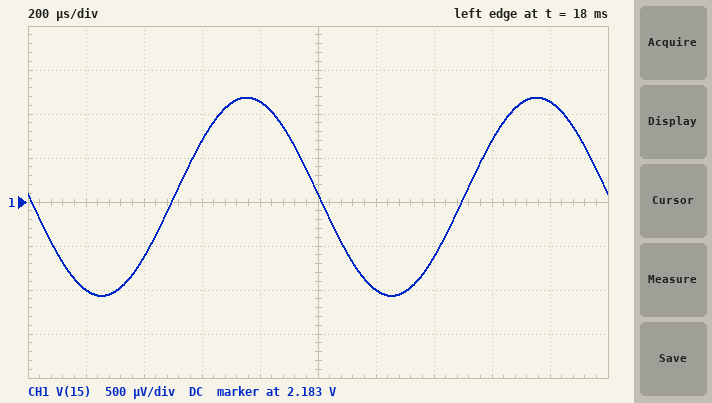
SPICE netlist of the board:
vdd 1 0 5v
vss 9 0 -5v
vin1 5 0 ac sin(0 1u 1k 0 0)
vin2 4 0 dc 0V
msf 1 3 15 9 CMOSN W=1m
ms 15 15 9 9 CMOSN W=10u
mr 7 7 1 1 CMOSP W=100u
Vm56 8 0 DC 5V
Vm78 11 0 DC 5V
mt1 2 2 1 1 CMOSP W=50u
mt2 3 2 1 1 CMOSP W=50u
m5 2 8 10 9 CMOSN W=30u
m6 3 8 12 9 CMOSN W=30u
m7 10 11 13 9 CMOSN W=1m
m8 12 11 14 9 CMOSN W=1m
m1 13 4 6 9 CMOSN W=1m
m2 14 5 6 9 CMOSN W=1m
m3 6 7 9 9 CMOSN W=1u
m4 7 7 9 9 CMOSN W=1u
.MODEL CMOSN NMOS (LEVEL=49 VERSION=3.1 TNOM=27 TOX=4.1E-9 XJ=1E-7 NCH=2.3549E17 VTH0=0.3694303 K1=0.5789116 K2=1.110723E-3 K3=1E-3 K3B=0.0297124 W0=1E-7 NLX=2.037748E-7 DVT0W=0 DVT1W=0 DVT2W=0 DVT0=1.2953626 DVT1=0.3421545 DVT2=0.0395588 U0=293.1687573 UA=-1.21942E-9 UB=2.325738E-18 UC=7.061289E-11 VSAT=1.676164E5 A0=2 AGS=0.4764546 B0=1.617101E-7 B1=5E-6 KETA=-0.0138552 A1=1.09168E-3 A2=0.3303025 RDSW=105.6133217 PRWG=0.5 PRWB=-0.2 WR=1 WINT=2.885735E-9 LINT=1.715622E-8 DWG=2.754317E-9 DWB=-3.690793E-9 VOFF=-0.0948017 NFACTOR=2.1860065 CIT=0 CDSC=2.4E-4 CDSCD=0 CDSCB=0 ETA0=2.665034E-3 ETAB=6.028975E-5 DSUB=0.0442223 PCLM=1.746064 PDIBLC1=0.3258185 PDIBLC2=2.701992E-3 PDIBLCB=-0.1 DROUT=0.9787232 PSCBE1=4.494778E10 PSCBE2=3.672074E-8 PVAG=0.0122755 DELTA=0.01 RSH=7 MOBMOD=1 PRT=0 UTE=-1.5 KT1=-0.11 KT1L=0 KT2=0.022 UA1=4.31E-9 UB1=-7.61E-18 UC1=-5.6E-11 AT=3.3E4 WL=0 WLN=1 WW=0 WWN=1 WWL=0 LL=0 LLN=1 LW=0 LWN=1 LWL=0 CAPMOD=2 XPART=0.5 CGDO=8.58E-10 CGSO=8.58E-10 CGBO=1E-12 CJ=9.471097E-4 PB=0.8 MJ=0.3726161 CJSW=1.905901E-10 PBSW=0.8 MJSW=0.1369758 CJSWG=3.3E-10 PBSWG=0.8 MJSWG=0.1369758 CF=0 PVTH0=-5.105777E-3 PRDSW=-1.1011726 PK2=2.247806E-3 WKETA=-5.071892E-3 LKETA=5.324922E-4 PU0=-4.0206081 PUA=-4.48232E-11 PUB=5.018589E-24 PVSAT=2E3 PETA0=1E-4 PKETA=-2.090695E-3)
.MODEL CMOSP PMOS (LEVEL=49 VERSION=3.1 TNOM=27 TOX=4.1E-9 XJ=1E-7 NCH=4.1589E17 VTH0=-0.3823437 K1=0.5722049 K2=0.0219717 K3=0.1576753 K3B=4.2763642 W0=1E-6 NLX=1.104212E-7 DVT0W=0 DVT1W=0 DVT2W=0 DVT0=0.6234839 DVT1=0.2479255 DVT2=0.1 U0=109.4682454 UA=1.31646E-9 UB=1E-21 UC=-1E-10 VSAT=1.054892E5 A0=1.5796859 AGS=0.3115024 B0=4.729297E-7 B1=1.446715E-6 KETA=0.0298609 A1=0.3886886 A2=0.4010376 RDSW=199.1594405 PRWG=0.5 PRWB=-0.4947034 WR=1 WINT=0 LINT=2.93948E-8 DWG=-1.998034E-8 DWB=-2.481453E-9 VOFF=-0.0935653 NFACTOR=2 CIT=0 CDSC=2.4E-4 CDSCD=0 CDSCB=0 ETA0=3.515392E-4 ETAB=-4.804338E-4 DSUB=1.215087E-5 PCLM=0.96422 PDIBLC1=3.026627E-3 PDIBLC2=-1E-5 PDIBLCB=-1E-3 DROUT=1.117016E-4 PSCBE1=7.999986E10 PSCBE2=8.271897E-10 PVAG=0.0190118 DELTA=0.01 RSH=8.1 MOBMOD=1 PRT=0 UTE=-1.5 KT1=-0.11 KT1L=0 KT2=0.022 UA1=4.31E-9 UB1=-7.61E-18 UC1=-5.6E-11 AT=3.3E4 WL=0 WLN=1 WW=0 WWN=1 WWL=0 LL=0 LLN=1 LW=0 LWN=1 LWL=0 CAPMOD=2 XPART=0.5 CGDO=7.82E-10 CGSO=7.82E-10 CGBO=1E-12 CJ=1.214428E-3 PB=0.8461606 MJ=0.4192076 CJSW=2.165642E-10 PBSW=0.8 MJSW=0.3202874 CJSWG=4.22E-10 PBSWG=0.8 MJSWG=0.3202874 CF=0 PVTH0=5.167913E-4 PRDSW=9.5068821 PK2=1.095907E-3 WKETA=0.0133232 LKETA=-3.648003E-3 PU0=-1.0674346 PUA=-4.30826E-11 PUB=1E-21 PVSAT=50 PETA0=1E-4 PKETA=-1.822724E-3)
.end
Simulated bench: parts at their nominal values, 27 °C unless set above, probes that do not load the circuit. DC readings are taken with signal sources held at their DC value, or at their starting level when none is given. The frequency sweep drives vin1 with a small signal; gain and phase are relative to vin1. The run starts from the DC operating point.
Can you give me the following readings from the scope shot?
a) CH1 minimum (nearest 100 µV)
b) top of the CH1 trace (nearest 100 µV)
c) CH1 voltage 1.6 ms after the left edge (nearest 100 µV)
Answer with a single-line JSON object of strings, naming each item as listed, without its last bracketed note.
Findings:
{"CH1 minimum": "2.1819 V", "top of the CH1 trace": "2.1842 V", "CH1 voltage 1.6 ms after the left edge": "2.1837 V"}
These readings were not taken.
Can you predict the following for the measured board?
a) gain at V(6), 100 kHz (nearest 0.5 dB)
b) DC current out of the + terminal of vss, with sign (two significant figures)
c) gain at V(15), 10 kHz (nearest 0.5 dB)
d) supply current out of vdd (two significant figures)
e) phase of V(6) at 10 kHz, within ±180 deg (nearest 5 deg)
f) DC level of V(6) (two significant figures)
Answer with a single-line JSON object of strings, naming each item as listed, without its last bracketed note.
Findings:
{"gain at V(6), 100 kHz": "-7.0 dB", "DC current out of the + terminal of vss, with sign": "-3.8 mA", "gain at V(15), 10 kHz": "60.5 dB", "supply current out of vdd": "3.8 mA", "phase of V(6) at 10 kHz, within ±180 deg": "0 deg", "DC level of V(6)": "-1.1 V"}
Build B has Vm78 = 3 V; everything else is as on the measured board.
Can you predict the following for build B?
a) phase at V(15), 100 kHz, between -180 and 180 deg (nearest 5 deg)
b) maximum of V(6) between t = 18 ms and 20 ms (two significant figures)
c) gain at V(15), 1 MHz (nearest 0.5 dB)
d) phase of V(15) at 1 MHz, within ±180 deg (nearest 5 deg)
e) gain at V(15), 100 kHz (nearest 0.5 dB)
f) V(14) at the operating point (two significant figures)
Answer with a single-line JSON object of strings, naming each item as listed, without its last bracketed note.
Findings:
{"phase at V(15), 100 kHz, between -180 and 180 deg": "110 deg", "maximum of V(6) between t = 18 ms and 20 ms": "-1.1 V", "gain at V(15), 1 MHz": "32.0 dB", "phase of V(15) at 1 MHz, within ±180 deg": "80 deg", "gain at V(15), 100 kHz": "51.5 dB", "V(14) at the operating point": "1.6 V"}
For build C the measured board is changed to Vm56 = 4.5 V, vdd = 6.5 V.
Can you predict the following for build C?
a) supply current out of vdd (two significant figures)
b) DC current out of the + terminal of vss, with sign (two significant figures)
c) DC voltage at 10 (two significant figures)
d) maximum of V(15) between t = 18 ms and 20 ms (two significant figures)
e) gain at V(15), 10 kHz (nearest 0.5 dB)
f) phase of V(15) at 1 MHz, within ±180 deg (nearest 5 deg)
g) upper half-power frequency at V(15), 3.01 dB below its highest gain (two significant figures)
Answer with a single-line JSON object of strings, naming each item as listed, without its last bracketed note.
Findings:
{"supply current out of vdd": "3.9 mA", "DC current out of the + terminal of vss, with sign": "-3.9 mA", "DC voltage at 10": "2.7 V", "maximum of V(15) between t = 18 ms and 20 ms": "3.6 V", "gain at V(15), 10 kHz": "60.0 dB", "phase of V(15) at 1 MHz, within ±180 deg": "50 deg", "upper half-power frequency at V(15), 3.01 dB below its highest gain": "33 kHz"}
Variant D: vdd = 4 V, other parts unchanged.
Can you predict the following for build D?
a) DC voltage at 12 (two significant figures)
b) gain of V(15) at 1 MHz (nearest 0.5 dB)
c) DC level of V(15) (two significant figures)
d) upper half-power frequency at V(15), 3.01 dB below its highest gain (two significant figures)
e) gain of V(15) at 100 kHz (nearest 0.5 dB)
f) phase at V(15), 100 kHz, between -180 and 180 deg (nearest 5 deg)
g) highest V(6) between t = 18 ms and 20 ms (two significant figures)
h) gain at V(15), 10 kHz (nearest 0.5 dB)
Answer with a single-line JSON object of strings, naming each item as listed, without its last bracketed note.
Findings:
{"DC voltage at 12": "2.9 V", "gain of V(15) at 1 MHz": "13.0 dB", "DC level of V(15)": "1.3 V", "upper half-power frequency at V(15), 3.01 dB below its highest gain": "14 kHz", "gain of V(15) at 100 kHz": "35.0 dB", "phase at V(15), 100 kHz, between -180 and 180 deg": "95 deg", "highest V(6) between t = 18 ms and 20 ms": "-1.1 V", "gain at V(15), 10 kHz": "50.5 dB"}
